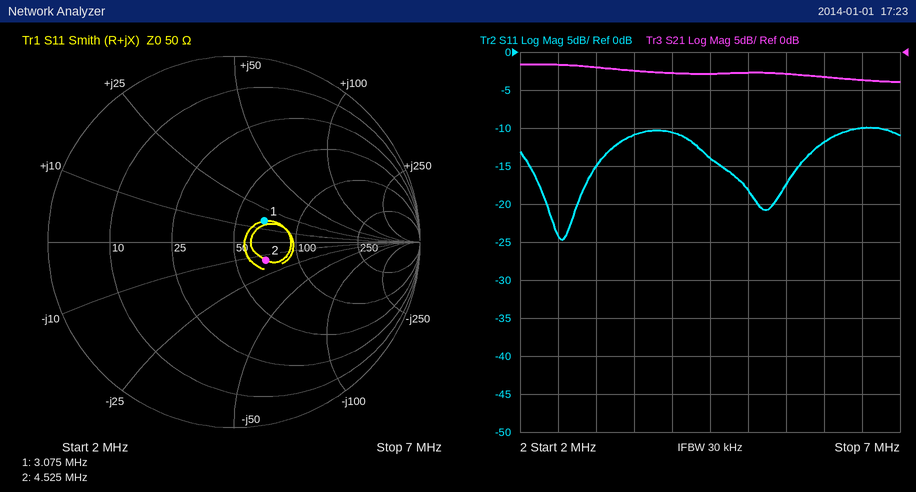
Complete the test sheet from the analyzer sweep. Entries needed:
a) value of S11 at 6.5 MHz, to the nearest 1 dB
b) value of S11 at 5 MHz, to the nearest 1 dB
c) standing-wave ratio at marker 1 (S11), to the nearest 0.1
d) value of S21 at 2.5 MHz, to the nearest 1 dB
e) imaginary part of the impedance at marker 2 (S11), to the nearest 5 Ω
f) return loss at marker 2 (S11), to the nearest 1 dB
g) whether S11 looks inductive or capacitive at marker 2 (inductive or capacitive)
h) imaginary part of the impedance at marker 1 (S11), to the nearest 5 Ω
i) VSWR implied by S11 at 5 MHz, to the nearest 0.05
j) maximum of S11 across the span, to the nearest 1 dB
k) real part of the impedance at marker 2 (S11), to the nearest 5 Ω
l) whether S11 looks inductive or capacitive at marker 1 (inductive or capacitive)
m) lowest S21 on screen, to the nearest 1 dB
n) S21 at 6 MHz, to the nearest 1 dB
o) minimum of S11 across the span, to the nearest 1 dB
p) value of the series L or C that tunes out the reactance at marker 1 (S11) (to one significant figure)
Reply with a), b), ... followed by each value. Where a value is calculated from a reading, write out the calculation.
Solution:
a) -10 dB
b) -18 dB
c) 1.5
d) -2 dB
e) -15 Ω
f) 14 dB
g) capacitive
h) +15 Ω
i) |Γ| = 10^(-18/20) = 0.1259; VSWR = (1 + 0.1259)/(1 − 0.1259) ≈ 1.29, so 1.30 to the nearest 0.05
j) -10 dB
k) 70 Ω
l) inductive
m) -4 dB
n) -3 dB
o) -25 dB
p) C = 1/(2π × 3.075 MHz × 15 Ω) ≈ 3 nF
